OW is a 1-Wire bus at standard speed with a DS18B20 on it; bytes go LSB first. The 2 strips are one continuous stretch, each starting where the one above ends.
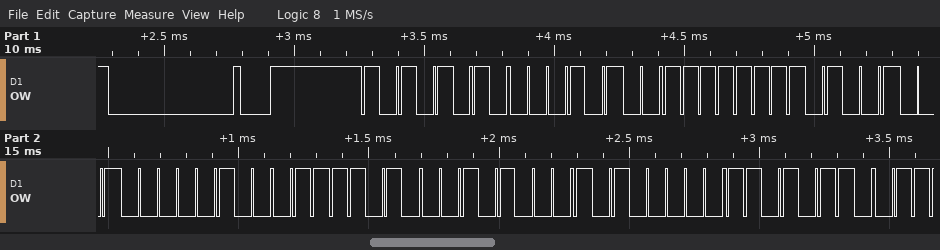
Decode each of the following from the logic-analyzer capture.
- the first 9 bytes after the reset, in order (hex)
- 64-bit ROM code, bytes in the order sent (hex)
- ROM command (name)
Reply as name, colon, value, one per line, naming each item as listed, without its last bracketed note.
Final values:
the first 9 bytes after the reset, in order: 55 28 FF 92 20 5E 14 05 6B
64-bit ROM code, bytes in the order sent: 28 FF 92 20 5E 14 05 6B
ROM command: Match ROM
